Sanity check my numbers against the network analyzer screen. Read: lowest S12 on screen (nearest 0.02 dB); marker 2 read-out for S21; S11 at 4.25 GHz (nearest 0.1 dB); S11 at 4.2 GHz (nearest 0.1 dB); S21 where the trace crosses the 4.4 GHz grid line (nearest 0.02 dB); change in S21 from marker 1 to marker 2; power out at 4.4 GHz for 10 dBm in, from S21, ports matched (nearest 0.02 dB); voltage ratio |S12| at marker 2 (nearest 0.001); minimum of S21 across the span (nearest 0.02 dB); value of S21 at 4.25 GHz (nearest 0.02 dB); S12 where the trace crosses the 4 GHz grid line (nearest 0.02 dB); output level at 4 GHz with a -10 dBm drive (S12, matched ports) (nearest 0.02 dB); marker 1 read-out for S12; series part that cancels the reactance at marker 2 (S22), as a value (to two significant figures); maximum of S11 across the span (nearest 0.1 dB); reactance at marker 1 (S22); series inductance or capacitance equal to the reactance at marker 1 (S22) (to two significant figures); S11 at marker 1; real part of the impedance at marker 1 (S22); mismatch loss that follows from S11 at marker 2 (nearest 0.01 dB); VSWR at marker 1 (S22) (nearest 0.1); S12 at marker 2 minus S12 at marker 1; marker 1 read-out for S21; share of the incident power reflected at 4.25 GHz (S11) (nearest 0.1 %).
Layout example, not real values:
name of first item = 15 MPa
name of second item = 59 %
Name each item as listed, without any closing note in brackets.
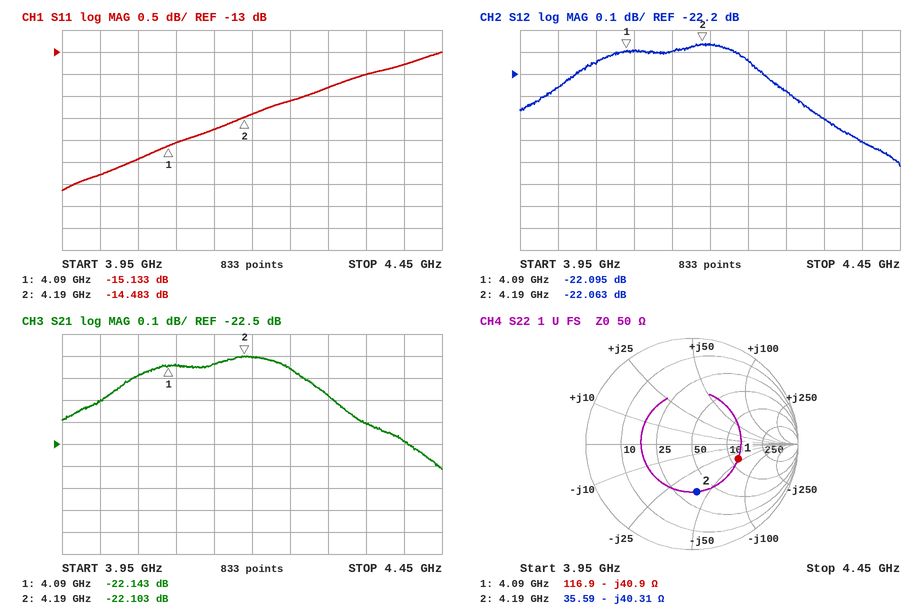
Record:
lowest S12 on screen = -22.62 dB
marker 2 read-out for S21 = -22.103 dB
S11 at 4.25 GHz = -14.1 dB
S11 at 4.2 GHz = -14.4 dB
S21 where the trace crosses the 4.4 GHz grid line = -22.48 dB
change in S21 from marker 1 to marker 2 = 0.040 dB
power out at 4.4 GHz for 10 dBm in, from S21, ports matched = -12.48 dBm
voltage ratio |S12| at marker 2 = 0.079
minimum of S21 across the span = -22.62 dB
value of S21 at 4.25 GHz = -22.16 dB
S12 where the trace crosses the 4 GHz grid line = -22.26 dB
output level at 4 GHz with a -10 dBm drive (S12, matched ports) = -32.26 dBm
marker 1 read-out for S12 = -22.095 dB
series part that cancels the reactance at marker 2 (S22), as a value = 1.5 nH
maximum of S11 across the span = -13.0 dB
reactance at marker 1 = -40.9 Ω
series inductance or capacitance equal to the reactance at marker 1 (S22) = 950 fF
S11 at marker 1 = -15.133 dB
real part of the impedance at marker 1 = 116.9 Ω
mismatch loss that follows from S11 at marker 2 = 0.16 dB
VSWR at marker 1 (S22) = 2.7
S12 at marker 2 minus S12 at marker 1 = 0.032 dB
marker 1 read-out for S21 = -22.143 dB
share of the incident power reflected at 4.25 GHz (S11) = 3.9 %
